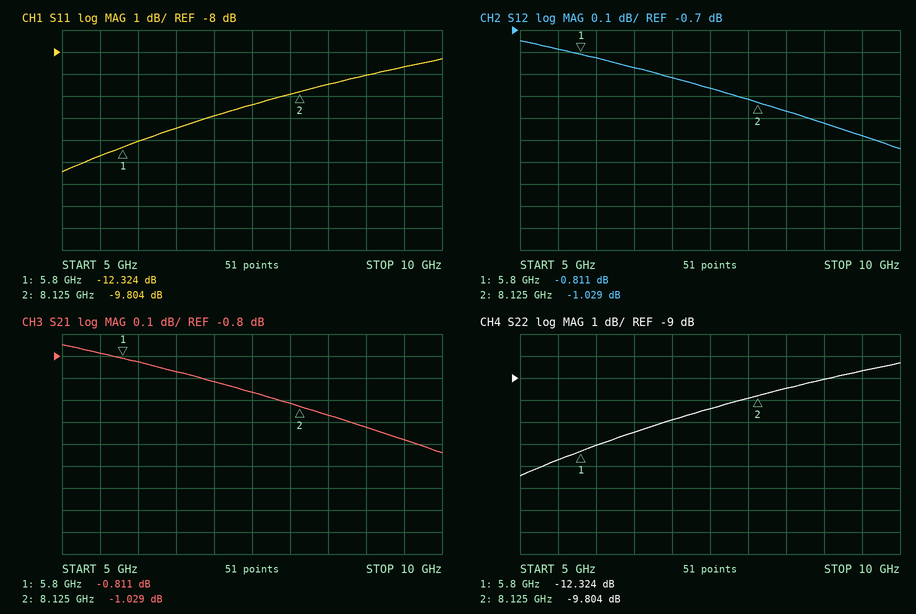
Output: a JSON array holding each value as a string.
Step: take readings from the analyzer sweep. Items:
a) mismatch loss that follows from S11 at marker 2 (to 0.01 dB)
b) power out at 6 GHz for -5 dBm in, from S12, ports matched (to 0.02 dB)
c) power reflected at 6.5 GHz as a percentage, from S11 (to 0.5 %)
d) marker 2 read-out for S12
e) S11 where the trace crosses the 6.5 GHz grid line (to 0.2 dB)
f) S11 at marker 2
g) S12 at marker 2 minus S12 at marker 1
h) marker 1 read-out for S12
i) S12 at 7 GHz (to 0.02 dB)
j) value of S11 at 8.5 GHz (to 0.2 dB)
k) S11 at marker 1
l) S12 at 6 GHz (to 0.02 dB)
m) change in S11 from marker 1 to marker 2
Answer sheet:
["0.48 dB", "-5.82 dBm", "7.0 %", "-1.029 dB", "-11.4 dB", "-9.804 dB", "-0.218 dB", "-0.811 dB", "-0.92 dB", "-9.4 dB", "-12.324 dB", "-0.82 dB", "2.520 dB"]
